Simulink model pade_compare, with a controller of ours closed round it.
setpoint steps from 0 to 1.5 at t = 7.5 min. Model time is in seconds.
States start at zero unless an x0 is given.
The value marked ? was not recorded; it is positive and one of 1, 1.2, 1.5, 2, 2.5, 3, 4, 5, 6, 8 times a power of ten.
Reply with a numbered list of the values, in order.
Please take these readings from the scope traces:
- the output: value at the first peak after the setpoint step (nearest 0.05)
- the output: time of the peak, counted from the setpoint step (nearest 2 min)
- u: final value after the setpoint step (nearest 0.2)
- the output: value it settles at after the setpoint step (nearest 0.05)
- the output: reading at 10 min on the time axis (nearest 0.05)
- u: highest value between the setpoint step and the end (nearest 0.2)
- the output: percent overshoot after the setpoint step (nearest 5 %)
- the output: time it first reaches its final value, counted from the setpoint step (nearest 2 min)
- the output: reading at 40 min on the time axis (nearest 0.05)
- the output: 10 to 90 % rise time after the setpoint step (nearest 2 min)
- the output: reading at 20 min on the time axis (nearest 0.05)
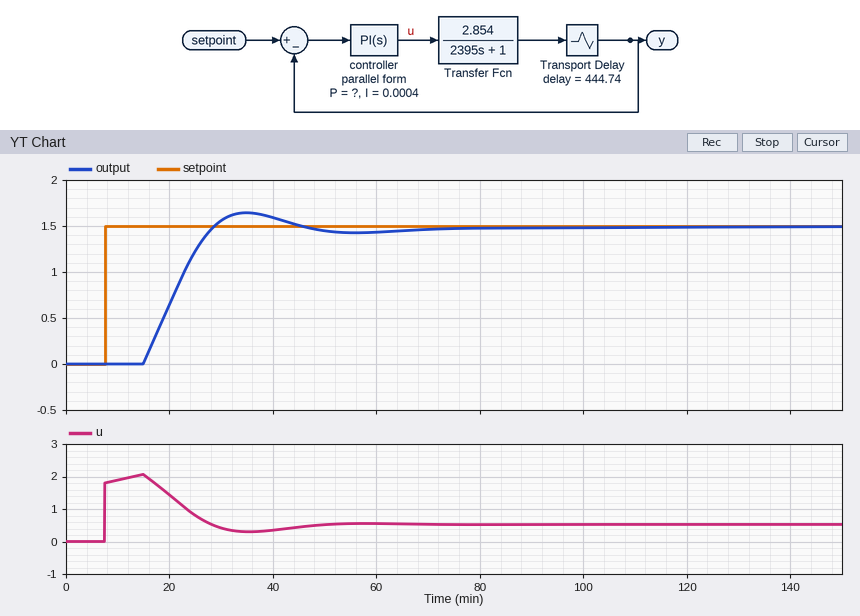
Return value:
1. 1.65
2. 28 min
3. 0.6
4. 1.50
5. 0.00
6. 2.0
7. 10 %
8. 22 min
9. 1.60
10. 10 min
11. 0.65
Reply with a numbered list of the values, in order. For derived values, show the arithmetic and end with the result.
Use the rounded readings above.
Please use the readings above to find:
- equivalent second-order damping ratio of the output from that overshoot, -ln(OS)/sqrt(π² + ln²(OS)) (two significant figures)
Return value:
1. ln(0.1) = -2.303; 2.303 / sqrt(9.870 + 5.302) = 0.59
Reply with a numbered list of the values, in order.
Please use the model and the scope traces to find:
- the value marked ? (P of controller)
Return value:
1. 1.2
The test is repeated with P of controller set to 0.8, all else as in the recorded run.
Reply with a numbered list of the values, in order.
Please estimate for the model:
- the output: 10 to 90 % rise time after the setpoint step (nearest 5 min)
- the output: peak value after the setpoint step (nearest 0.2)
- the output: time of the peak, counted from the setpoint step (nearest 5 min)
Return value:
1. 15 min
2. 1.6
3. 45 min
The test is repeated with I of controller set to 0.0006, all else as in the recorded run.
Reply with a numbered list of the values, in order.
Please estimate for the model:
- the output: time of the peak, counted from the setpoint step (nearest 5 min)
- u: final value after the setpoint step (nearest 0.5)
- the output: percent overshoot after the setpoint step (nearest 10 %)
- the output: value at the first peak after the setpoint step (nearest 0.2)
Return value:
1. 30 min
2. 0.5
3. 20 %
4. 1.8
